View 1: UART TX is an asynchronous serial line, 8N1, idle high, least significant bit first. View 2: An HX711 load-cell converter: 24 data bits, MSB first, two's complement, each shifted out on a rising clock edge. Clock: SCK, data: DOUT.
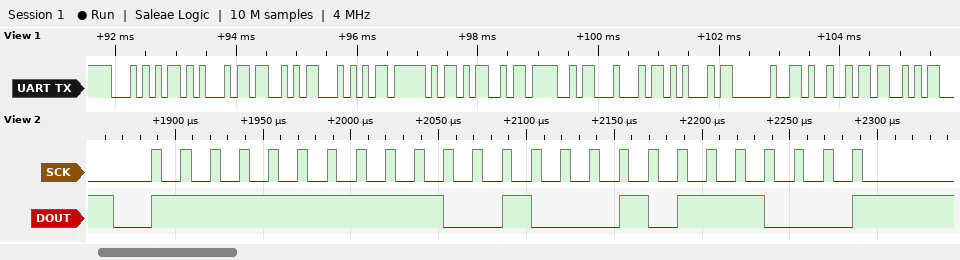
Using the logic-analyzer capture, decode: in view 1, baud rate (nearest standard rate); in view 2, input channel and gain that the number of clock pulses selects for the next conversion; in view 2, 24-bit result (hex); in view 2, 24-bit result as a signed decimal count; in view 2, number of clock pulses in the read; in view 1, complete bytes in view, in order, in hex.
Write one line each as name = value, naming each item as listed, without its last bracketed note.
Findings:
in view 1, baud rate = 9600 baud
in view 2, input channel and gain that the number of clock pulses selects for the next conversion = channel A, gain 128
in view 2, 24-bit result = 0xFFC8B8
in view 2, 24-bit result as a signed decimal count = -14152
in view 2, number of clock pulses in the read = 25
in view 1, complete bytes in view, in order, in hex = 54 45 53 54 5F 4D 4F 44 45 20 49 53
